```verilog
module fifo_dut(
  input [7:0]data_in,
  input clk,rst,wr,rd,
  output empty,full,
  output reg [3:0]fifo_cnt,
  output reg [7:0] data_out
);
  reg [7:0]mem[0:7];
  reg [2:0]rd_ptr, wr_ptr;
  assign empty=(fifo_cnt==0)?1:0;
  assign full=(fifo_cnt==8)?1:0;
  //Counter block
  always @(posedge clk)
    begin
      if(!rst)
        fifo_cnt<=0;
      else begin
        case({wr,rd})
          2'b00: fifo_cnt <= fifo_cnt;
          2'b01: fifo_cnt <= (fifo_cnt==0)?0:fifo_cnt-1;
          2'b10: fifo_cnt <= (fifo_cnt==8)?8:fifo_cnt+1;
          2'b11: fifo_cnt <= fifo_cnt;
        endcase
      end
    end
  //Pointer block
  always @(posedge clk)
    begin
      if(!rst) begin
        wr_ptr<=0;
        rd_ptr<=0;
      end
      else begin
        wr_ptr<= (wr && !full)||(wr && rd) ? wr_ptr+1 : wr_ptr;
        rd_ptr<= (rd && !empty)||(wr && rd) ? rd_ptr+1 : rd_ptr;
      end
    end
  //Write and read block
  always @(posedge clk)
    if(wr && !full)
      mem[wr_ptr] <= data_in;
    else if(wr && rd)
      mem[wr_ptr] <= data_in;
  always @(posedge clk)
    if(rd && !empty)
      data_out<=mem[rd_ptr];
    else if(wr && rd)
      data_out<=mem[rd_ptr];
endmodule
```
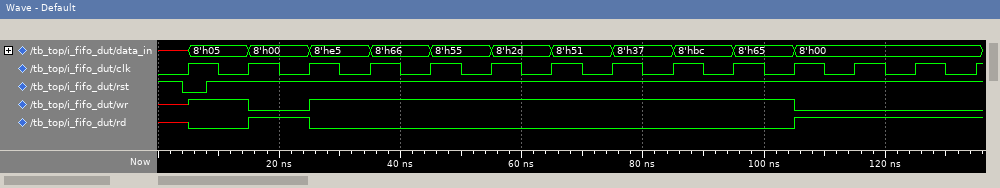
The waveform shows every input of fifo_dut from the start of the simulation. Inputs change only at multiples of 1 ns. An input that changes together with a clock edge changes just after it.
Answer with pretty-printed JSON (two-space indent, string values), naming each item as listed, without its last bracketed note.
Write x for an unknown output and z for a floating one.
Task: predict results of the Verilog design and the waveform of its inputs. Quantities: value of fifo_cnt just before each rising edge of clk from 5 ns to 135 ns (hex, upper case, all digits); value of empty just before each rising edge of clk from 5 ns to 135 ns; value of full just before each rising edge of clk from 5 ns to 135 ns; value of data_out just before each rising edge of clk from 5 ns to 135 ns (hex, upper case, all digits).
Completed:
{
  "value of fifo_cnt just before each rising edge of clk from 5 ns to 135 ns": "x, 0, 1, 0, 1, 2, 3, 4, 5, 6, 7, 8, 7, 6",
  "value of empty just before each rising edge of clk from 5 ns to 135 ns": "x 1 0 1 0 0 0 0 0 0 0 0 0 0",
  "value of full just before each rising edge of clk from 5 ns to 135 ns": "x 0 0 0 0 0 0 0 0 0 0 1 0 0",
  "value of data_out just before each rising edge of clk from 5 ns to 135 ns": "x, x, x, 05, 05, 05, 05, 05, 05, 05, 05, 05, E5, 66"
}
